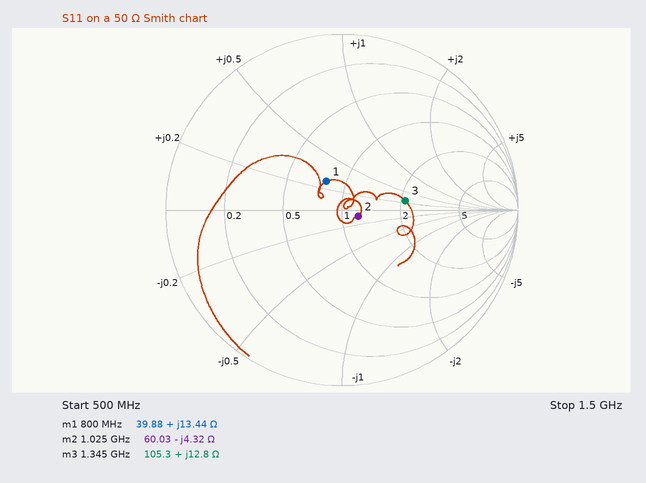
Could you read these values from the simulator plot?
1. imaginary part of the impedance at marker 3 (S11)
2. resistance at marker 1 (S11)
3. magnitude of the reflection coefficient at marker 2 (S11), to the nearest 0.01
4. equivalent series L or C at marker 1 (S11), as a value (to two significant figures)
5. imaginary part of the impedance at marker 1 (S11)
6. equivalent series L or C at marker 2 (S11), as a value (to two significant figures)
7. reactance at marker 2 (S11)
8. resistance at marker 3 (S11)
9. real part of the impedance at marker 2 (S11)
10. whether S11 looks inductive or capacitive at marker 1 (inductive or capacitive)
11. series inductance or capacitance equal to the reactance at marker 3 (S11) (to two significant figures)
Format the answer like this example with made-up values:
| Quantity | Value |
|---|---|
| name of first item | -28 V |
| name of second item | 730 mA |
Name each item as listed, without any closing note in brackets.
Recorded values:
| Quantity | Value |
|---|---|
| imaginary part of the impedance at marker 3 | +12.8 Ω |
| resistance at marker 1 | 39.88 Ω |
| magnitude of the reflection coefficient at marker 2 (S11), to the nearest 0.01 | 0.10 |
| equivalent series L or C at marker 1 (S11), as a value | 2.7 nH |
| imaginary part of the impedance at marker 1 | +13.44 Ω |
| equivalent series L or C at marker 2 (S11), as a value | 36 pF |
| reactance at marker 2 | -4.32 Ω |
| resistance at marker 3 | 105.3 Ω |
| real part of the impedance at marker 2 | 60.03 Ω |
| whether S11 looks inductive or capacitive at marker 1 | inductive |
| series inductance or capacitance equal to the reactance at marker 3 (S11) | 1.5 nH |
